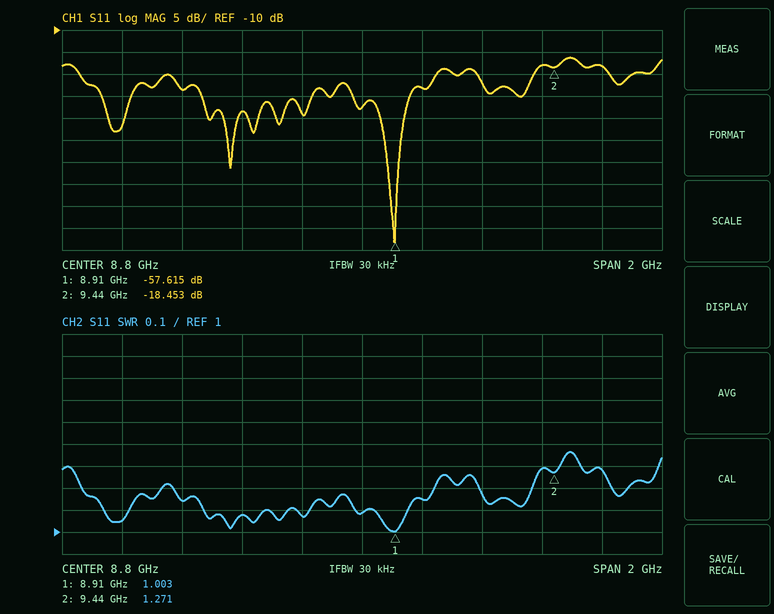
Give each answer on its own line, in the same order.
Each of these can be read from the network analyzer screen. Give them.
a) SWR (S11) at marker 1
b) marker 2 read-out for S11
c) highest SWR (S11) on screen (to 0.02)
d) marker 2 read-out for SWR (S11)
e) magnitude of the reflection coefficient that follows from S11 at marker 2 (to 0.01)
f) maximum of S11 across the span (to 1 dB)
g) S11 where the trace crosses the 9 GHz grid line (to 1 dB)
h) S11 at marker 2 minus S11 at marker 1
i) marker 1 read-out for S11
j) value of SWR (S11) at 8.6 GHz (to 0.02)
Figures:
1.003
-18.453 dB
1.36
1.271
0.12
-16 dB
-23 dB
39.162 dB
-57.615 dB
1.08
